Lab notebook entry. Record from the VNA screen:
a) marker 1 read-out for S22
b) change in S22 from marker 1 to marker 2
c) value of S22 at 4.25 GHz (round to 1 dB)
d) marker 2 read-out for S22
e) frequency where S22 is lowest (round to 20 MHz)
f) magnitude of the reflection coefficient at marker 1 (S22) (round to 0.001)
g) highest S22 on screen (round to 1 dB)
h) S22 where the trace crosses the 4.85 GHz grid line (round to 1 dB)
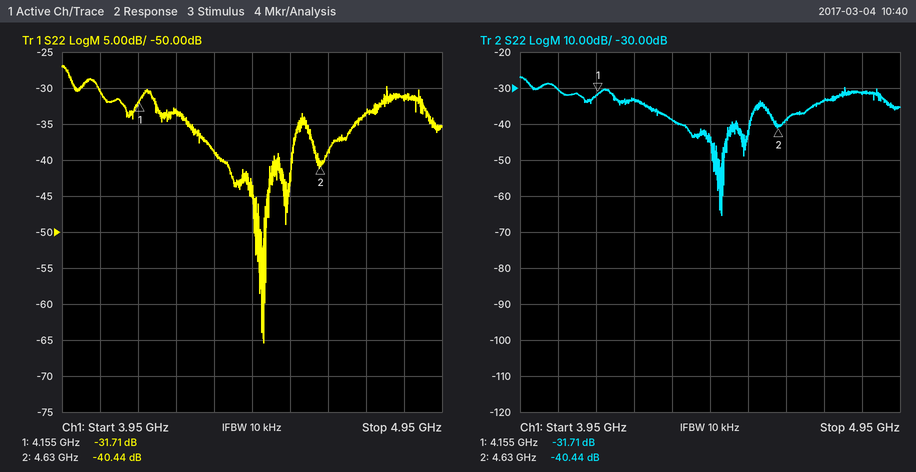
-31.71 dB
-8.73 dB
-33 dB
-40.44 dB
4.48 GHz
0.026
-27 dB
-31 dB
